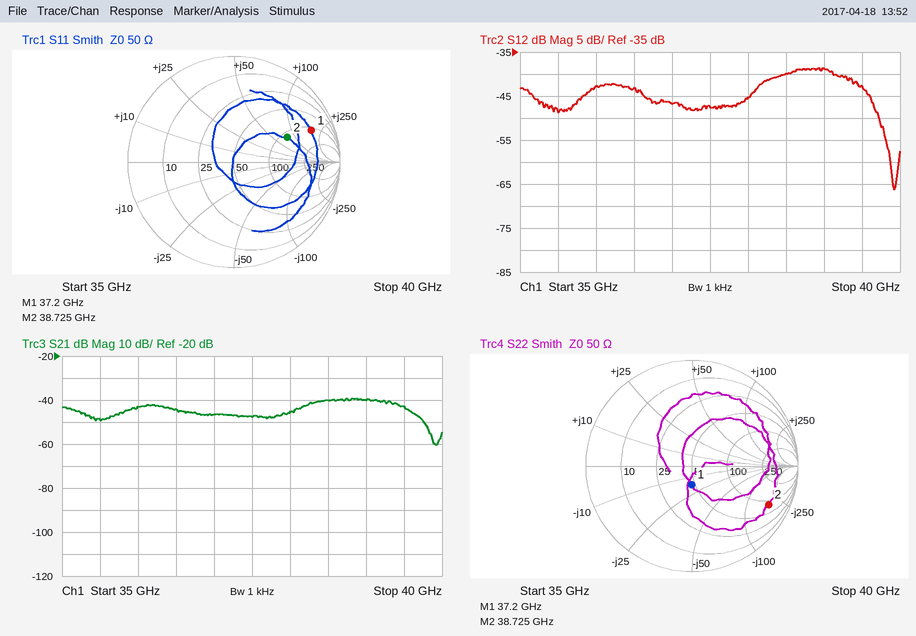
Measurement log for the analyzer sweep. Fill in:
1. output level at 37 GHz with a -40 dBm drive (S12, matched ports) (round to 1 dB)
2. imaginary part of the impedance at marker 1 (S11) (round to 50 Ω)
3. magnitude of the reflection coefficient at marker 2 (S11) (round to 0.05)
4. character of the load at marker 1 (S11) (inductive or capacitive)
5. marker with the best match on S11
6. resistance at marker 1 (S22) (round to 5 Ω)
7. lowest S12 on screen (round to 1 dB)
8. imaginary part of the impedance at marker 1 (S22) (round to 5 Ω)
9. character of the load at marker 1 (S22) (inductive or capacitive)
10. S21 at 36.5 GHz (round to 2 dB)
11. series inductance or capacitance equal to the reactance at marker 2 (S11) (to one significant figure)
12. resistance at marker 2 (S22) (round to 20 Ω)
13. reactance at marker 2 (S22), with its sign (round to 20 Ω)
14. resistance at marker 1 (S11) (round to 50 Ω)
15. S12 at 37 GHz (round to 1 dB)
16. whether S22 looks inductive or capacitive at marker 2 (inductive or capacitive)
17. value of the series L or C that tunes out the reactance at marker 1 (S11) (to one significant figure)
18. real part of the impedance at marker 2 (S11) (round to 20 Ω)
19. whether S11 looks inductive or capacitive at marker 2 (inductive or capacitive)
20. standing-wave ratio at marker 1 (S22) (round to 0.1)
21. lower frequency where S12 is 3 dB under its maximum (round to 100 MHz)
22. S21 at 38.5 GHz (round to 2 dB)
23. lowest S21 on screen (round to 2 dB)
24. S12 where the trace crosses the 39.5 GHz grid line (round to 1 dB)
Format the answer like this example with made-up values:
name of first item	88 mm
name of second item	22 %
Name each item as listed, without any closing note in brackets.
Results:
output level at 37 GHz with a -40 dBm drive (S12, matched ports)	-87 dBm
imaginary part of the impedance at marker 1 (S11)	+200 Ω
magnitude of the reflection coefficient at marker 2 (S11)	0.55
character of the load at marker 1 (S11)	inductive
marker with the best match on S11	marker 2
resistance at marker 1 (S22)	45 Ω
lowest S12 on screen	-66 dB
imaginary part of the impedance at marker 1 (S22)	-15 Ω
character of the load at marker 1 (S22)	capacitive
S21 at 36.5 GHz	-44 dB
series inductance or capacitance equal to the reactance at marker 2 (S11)	300 pH
resistance at marker 2 (S22)	80 Ω
reactance at marker 2 (S22), with its sign	-180 Ω
resistance at marker 1 (S11)	100 Ω
S12 at 37 GHz	-47 dB
whether S22 looks inductive or capacitive at marker 2	capacitive
value of the series L or C that tunes out the reactance at marker 1 (S11)	20 fF
real part of the impedance at marker 2 (S11)	120 Ω
whether S11 looks inductive or capacitive at marker 2	inductive
standing-wave ratio at marker 1 (S22)	1.4
lower frequency where S12 is 3 dB under its maximum	38.2 GHz
S21 at 38.5 GHz	-40 dB
lowest S21 on screen	-60 dB
S12 where the trace crosses the 39.5 GHz grid line	-43 dB
